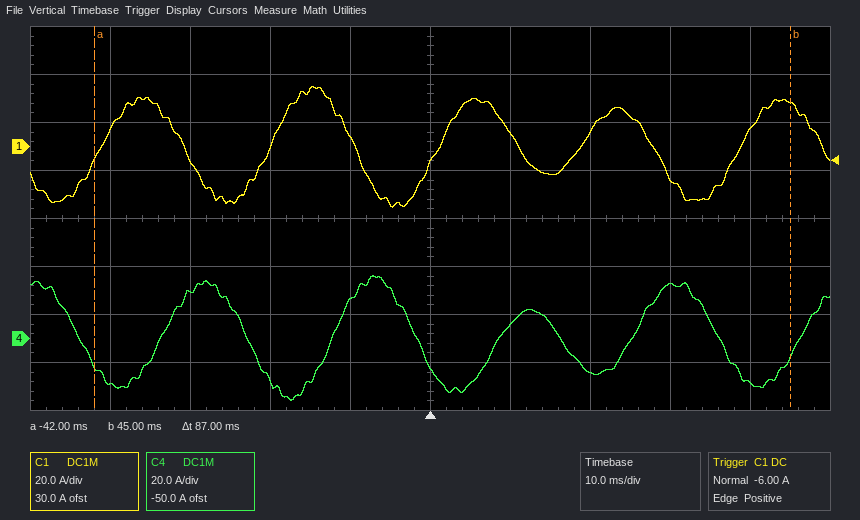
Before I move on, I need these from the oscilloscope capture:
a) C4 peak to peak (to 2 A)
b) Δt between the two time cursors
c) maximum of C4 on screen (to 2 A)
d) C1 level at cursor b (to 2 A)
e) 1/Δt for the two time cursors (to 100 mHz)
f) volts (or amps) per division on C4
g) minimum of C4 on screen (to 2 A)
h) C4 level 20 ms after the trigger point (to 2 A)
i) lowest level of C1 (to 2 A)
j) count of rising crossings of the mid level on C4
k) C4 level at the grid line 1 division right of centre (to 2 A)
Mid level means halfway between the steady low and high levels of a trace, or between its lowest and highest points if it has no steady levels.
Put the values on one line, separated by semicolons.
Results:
52 A; 87 ms; 26 A; 18 A; 11.5 Hz; 20 A; -26 A; -14 A; -26 A; 5; 6 A
